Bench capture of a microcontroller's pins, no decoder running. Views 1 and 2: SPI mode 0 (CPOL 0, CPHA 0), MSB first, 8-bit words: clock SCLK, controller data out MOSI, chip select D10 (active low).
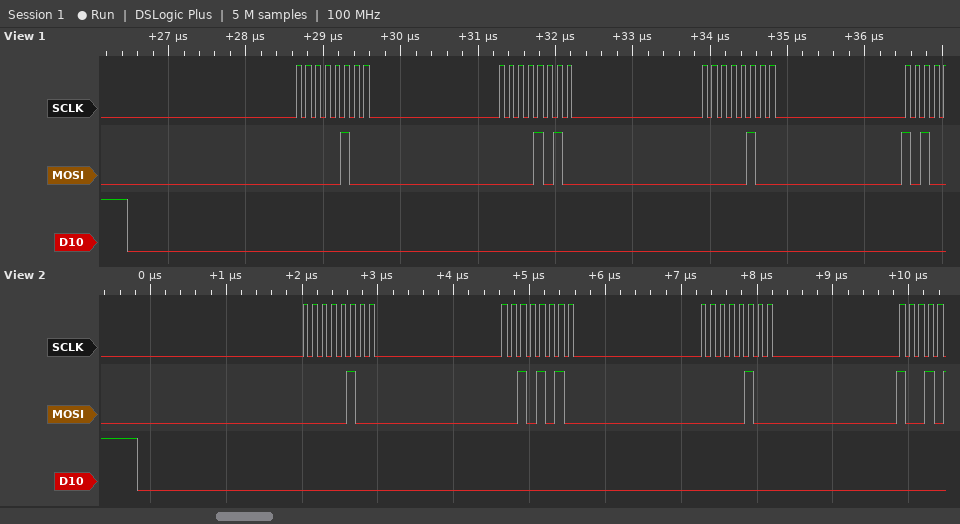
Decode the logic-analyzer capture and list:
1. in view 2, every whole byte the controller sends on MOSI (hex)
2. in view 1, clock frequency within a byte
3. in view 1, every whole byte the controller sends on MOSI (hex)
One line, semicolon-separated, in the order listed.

04 2A 04; 8 MHz; 04 0A 04
